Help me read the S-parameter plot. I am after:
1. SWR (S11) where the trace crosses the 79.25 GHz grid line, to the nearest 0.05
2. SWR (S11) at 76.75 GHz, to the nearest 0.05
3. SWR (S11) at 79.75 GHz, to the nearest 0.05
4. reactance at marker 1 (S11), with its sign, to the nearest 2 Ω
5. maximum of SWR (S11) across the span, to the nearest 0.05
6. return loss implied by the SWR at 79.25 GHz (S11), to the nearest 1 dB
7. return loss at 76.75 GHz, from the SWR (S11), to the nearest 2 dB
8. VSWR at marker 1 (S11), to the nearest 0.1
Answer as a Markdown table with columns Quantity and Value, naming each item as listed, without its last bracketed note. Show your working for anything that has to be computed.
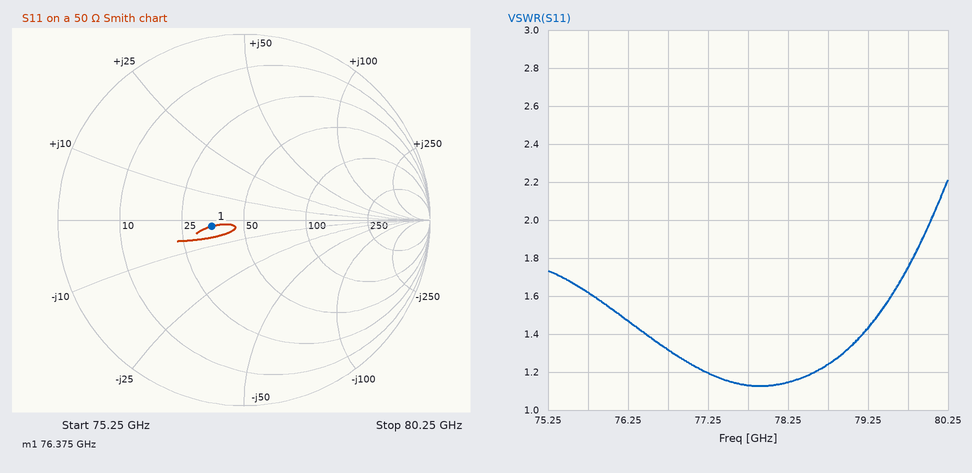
| Quantity | Value |
|---|---|
| SWR (S11) where the trace crosses the 79.25 GHz grid line, to the nearest 0.05 | 1.45 |
| SWR (S11) at 76.75 GHz, to the nearest 0.05 | 1.30 |
| SWR (S11) at 79.75 GHz, to the nearest 0.05 | 1.75 |
| reactance at marker 1 (S11), with its sign, to the nearest 2 Ω | -2 Ω |
| maximum of SWR (S11) across the span, to the nearest 0.05 | 2.20 |
| return loss implied by the SWR at 79.25 GHz (S11), to the nearest 1 dB | −20 log10((1.45 − 1)/(1.45 + 1)) ≈ 15 dB |
| return loss at 76.75 GHz, from the SWR (S11), to the nearest 2 dB | −20 log10((1.3 − 1)/(1.3 + 1)) ≈ 18 dB |
| VSWR at marker 1 (S11), to the nearest 0.1 | 1.4 |
